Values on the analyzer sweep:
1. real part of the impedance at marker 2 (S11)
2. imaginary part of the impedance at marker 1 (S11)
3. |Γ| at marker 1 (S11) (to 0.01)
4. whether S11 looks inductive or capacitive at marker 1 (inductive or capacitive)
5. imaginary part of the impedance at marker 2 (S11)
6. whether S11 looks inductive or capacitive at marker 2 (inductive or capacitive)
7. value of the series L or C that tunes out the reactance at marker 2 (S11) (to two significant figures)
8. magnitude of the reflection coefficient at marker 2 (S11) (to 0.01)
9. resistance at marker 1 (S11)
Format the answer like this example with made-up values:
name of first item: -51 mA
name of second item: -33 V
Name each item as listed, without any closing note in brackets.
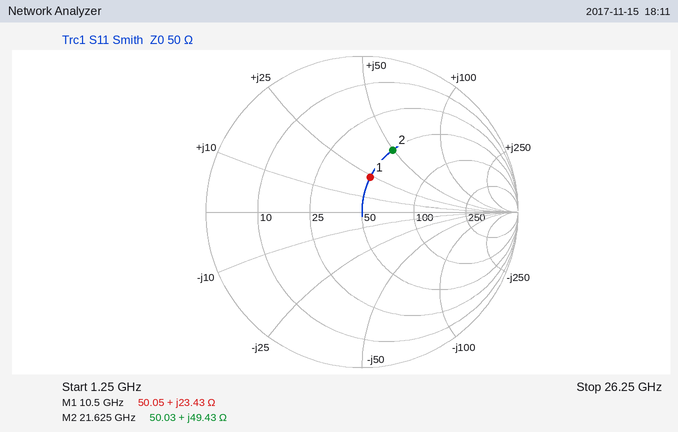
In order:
real part of the impedance at marker 2: 50.03 Ω
imaginary part of the impedance at marker 1: +23.43 Ω
|Γ| at marker 1 (S11): 0.23
whether S11 looks inductive or capacitive at marker 1: inductive
imaginary part of the impedance at marker 2: +49.43 Ω
whether S11 looks inductive or capacitive at marker 2: inductive
value of the series L or C that tunes out the reactance at marker 2 (S11): 150 fF
magnitude of the reflection coefficient at marker 2 (S11): 0.44
resistance at marker 1: 50.05 Ω
